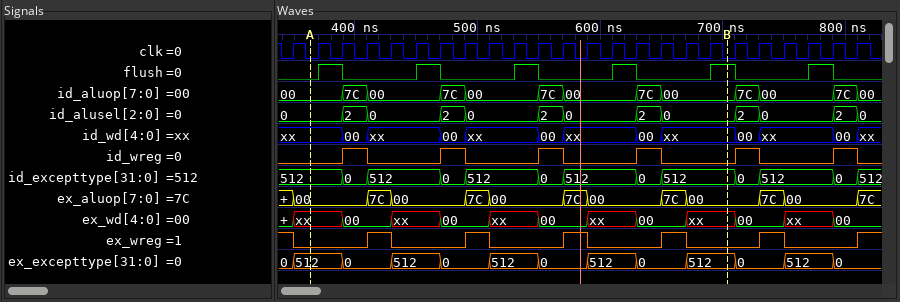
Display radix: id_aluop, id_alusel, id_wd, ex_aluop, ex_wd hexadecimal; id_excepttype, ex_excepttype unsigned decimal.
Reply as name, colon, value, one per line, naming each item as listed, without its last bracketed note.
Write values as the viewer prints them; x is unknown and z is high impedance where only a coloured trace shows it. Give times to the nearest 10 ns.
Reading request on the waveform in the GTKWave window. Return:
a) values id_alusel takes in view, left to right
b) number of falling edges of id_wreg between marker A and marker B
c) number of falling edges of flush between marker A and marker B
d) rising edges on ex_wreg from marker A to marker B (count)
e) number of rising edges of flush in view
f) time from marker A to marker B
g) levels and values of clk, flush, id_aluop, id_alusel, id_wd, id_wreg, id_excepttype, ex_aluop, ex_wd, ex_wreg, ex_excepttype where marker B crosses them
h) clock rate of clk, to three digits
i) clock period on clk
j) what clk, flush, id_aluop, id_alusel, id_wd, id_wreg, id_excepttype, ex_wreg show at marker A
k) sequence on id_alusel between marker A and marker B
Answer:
values id_alusel takes in view, left to right: 0, 2, 0, 2, 0, 2, 0, 2, 0, 2, 0, 2, 0
number of falling edges of id_wreg between marker A and marker B: 4
number of falling edges of flush between marker A and marker B: 4
rising edges on ex_wreg from marker A to marker B: 4
number of rising edges of flush in view: 6
time from marker A to marker B: 340 ns
levels and values of clk, flush, id_aluop, id_alusel, id_wd, id_wreg, id_excepttype, ex_aluop, ex_wd, ex_wreg, ex_excepttype where marker B crosses them: clk=0, flush=1, id_aluop=00, id_alusel=0, id_wd=xx, id_wreg=0, id_excepttype=512, ex_aluop=00, ex_wd=xx, ex_wreg=0, ex_excepttype=512
clock rate of clk, to three digits: 50.0 MHz
clock period on clk: 20 ns
what clk, flush, id_aluop, id_alusel, id_wd, id_wreg, id_excepttype, ex_wreg show at marker A: clk=0, flush=0, id_aluop=00, id_alusel=0, id_wd=xx, id_wreg=0, id_excepttype=512, ex_wreg=0
sequence on id_alusel between marker A and marker B: 0, 2, 0, 2, 0, 2, 0, 2, 0
